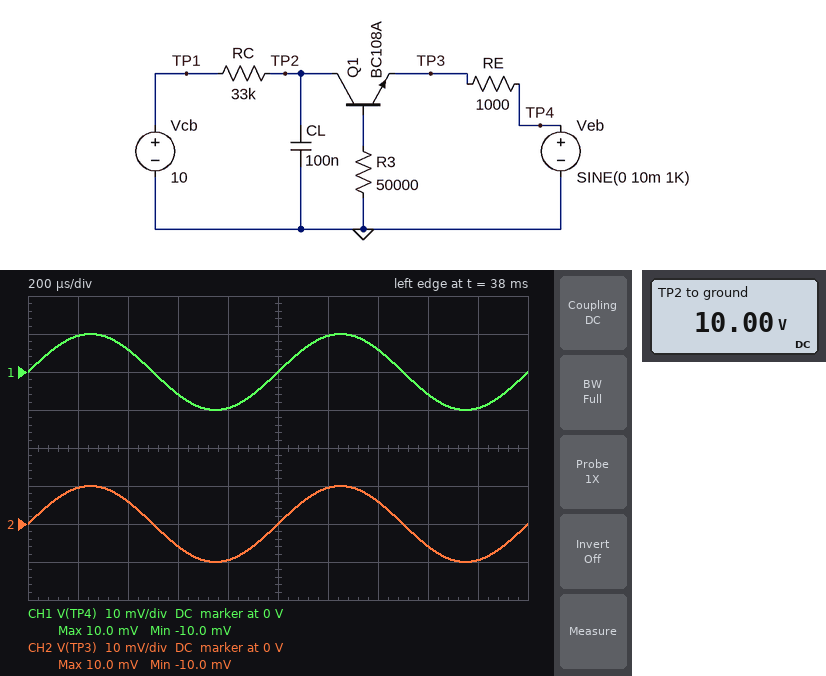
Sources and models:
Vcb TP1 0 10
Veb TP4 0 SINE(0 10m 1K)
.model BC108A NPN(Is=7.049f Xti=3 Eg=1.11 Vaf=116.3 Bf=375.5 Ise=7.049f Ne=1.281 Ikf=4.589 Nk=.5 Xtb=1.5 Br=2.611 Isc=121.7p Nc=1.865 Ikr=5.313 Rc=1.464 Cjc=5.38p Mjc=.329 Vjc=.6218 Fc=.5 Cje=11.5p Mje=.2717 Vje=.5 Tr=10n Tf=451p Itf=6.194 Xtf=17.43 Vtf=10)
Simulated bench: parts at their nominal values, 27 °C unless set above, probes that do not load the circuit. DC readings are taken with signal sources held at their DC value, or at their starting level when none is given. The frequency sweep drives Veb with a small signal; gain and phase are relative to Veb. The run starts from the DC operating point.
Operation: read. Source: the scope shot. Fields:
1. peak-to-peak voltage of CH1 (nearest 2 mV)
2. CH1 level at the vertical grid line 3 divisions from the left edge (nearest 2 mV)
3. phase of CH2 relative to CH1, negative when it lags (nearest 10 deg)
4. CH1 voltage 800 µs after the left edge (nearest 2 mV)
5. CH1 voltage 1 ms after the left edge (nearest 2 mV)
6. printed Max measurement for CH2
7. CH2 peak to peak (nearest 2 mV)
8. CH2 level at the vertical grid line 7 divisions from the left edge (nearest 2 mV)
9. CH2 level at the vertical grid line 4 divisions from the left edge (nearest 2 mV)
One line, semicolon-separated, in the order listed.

20 mV; -6 mV; 0 deg; -10 mV; 0 V; 10.0 mV; 20 mV; 6 mV; -10 mV
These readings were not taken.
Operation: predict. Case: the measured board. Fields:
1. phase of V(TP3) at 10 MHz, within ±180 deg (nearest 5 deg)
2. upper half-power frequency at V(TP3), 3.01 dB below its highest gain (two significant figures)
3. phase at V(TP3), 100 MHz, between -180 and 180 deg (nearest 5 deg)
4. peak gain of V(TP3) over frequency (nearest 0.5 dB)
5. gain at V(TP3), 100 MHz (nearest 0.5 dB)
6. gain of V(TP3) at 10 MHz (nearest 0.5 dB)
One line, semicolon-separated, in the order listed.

-5 deg; 88 MHz; -50 deg; 0 dB; -3.5 dB; 0 dB
